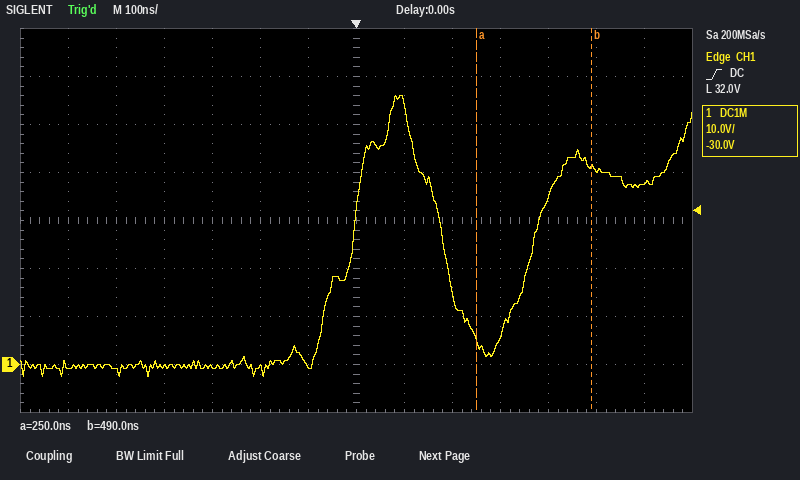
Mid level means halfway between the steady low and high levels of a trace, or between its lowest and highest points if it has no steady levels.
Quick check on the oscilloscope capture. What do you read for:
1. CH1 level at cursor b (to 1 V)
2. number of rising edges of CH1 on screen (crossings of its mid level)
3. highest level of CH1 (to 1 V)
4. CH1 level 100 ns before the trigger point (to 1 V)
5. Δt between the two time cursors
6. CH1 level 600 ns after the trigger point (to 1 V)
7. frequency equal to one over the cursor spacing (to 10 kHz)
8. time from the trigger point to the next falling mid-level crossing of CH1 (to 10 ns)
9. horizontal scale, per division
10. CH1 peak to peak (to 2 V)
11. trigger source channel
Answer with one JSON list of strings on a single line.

["41 V", "2", "56 V", "0 V", "240 ns", "38 V", "4.17 MHz", "180 ns", "100 ns", "58 V", "CH1"]
